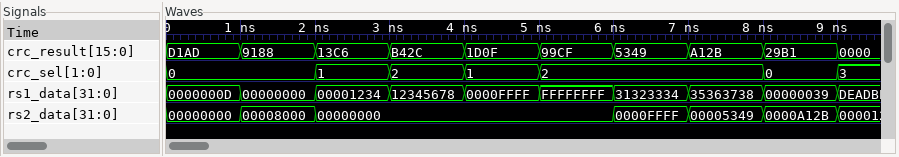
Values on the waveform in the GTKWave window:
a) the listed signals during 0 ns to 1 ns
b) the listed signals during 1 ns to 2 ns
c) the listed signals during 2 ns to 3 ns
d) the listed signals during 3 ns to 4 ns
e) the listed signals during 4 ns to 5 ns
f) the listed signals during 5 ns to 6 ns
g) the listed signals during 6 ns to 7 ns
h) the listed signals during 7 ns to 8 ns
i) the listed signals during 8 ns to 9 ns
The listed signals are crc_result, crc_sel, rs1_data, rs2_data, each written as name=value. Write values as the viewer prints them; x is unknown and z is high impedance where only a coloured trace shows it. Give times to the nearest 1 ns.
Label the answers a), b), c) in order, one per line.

a) crc_result=D1AD, crc_sel=0, rs1_data=0000000D, rs2_data=00000000
b) crc_result=9188, crc_sel=0, rs1_data=00000000, rs2_data=00008000
c) crc_result=13C6, crc_sel=1, rs1_data=00001234, rs2_data=00000000
d) crc_result=B42C, crc_sel=2, rs1_data=12345678, rs2_data=00000000
e) crc_result=1D0F, crc_sel=1, rs1_data=0000FFFF, rs2_data=00000000
f) crc_result=99CF, crc_sel=2, rs1_data=FFFFFFFF, rs2_data=00000000
g) crc_result=5349, crc_sel=2, rs1_data=31323334, rs2_data=0000FFFF
h) crc_result=A12B, crc_sel=2, rs1_data=35363738, rs2_data=00005349
i) crc_result=29B1, crc_sel=0, rs1_data=00000039, rs2_data=0000A12B
